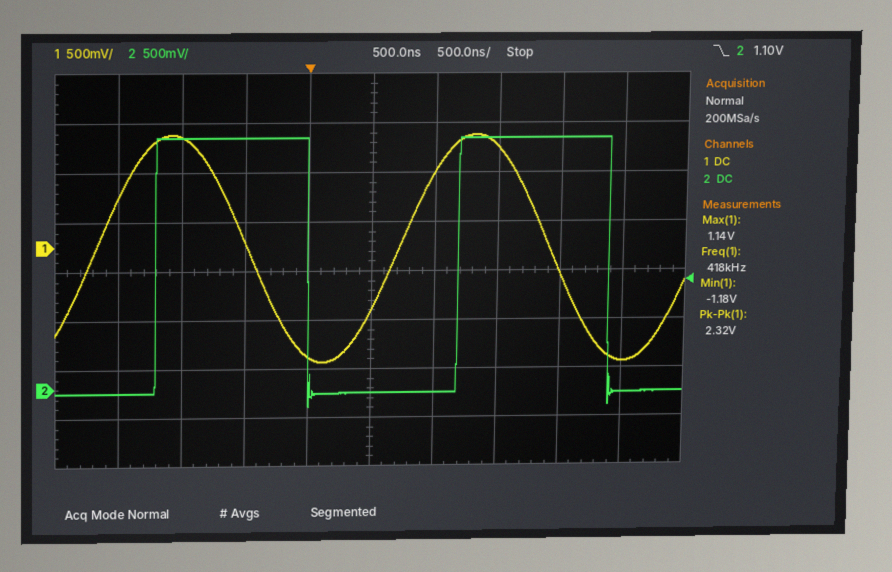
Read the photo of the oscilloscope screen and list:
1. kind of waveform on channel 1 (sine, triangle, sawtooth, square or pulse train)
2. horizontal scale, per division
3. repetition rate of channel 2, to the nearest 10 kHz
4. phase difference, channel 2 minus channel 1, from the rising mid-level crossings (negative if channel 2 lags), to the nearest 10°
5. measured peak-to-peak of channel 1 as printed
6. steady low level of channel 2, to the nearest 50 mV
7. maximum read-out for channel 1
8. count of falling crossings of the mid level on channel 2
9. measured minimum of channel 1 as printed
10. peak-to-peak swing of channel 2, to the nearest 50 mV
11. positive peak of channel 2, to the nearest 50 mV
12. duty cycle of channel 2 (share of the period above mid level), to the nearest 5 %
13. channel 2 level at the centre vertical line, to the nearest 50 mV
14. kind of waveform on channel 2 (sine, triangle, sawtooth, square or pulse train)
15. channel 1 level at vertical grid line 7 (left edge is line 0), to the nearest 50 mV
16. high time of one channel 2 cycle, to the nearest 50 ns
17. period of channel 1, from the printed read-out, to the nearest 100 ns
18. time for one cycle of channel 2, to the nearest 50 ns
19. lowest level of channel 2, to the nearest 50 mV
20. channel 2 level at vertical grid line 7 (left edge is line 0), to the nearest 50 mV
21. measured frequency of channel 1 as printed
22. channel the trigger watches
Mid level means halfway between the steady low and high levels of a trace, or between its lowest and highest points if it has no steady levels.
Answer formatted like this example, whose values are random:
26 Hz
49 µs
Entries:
sine
500 ns
420 kHz
-70°
2.32 V
-50 mV
1.14 V
2
-1.18 V
2.75 V
2.55 V
50 %
-50 mV
square
1.00 V
1.20 µs
2.4 µs
2.40 µs
-200 mV
2.55 V
418 kHz
channel 2
